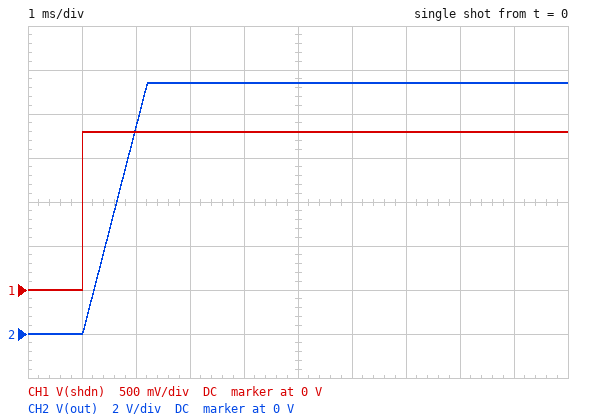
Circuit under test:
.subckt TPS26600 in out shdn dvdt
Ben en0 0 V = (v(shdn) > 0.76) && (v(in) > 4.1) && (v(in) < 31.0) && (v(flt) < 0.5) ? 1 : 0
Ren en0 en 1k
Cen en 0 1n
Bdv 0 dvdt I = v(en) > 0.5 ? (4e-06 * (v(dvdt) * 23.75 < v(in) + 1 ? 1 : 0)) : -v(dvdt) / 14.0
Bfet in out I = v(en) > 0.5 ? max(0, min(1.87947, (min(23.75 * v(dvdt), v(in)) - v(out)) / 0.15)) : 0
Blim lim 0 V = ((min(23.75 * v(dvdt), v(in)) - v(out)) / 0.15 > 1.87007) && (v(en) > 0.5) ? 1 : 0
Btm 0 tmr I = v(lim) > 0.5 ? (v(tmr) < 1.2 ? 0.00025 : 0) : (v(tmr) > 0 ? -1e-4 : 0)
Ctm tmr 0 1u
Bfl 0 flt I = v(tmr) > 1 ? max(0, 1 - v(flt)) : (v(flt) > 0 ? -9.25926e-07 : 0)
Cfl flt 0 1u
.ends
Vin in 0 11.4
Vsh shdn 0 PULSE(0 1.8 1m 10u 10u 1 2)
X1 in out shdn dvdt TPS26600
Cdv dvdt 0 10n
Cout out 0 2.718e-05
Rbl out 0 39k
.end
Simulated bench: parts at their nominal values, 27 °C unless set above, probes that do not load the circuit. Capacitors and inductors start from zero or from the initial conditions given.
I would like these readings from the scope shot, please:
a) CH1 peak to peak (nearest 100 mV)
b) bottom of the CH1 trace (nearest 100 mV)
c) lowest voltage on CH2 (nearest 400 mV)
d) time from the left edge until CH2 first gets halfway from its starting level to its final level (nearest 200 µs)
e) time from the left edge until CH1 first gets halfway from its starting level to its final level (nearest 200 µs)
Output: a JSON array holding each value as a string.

["1.8 V", "0 V", "0 V", "1.6 ms", "1.0 ms"]
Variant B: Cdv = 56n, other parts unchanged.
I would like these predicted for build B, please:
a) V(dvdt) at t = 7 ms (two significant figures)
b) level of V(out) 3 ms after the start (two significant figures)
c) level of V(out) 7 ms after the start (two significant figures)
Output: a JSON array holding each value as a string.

["430 mV", "3.4 V", "10 V"]
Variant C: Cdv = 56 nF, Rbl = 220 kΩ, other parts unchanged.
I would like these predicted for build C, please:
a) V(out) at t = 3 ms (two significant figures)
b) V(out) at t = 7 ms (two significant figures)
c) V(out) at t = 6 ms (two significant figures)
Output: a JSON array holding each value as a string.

["3.4 V", "10 V", "8.5 V"]
